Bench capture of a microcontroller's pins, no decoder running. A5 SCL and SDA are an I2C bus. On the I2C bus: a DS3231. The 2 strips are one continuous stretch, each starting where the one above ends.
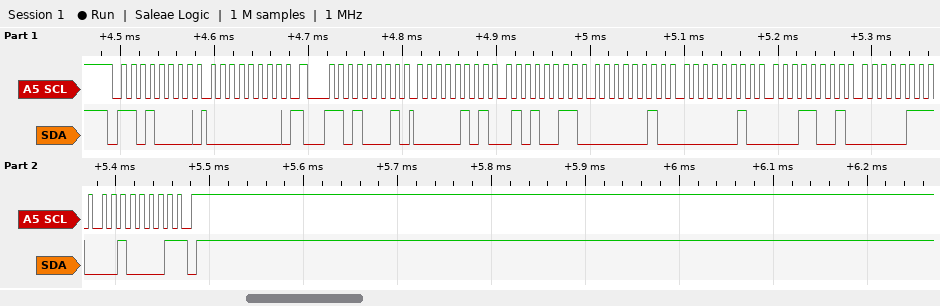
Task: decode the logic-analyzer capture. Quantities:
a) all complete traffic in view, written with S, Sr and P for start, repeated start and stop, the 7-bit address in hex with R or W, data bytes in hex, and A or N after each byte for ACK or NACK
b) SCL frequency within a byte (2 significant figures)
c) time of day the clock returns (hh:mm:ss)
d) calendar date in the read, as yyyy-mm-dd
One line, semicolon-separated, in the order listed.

S 68W A 00 A Sr 68R A 05 A 53 A 02 A 02 A 19 A 07 A 21 N P; 100 kHz; 02:53:05; 2021-07-19
